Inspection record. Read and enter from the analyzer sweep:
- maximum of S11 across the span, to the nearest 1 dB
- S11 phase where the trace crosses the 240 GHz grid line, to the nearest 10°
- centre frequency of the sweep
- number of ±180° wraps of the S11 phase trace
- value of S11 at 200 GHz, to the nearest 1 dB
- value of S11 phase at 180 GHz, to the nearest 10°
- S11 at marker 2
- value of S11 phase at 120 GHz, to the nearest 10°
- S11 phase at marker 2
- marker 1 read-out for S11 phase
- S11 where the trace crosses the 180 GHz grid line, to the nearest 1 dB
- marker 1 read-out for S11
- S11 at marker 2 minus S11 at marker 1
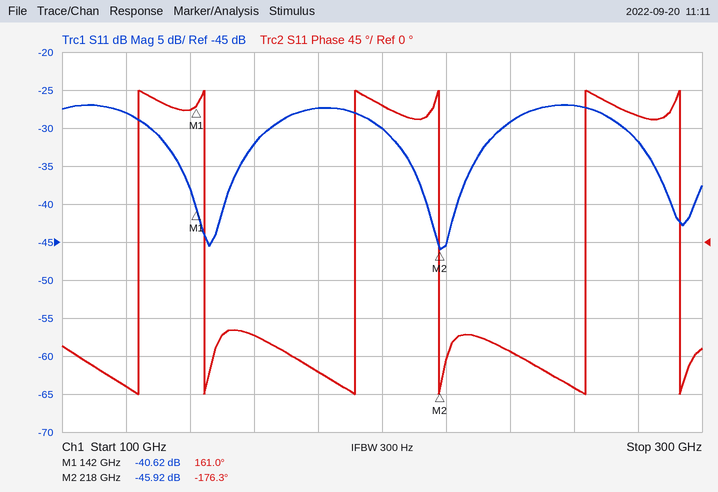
-27 dB
-130°
200 GHz
6
-30 dB
-150°
-45.92 dB
-170°
-176.3°
161.0°
-27 dB
-40.62 dB
-5.30 dB
